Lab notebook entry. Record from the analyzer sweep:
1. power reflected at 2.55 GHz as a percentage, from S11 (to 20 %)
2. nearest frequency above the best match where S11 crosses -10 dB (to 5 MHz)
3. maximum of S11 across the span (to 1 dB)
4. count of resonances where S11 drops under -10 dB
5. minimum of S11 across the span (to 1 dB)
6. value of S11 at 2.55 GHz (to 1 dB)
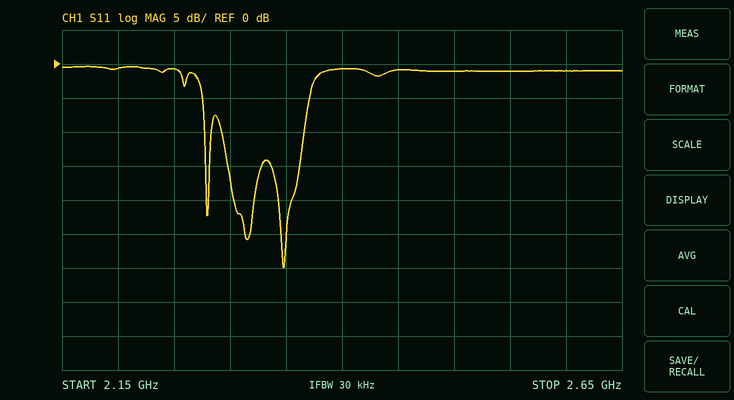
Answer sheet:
80 %
2.365 GHz
0 dB
3
-30 dB
-1 dB
